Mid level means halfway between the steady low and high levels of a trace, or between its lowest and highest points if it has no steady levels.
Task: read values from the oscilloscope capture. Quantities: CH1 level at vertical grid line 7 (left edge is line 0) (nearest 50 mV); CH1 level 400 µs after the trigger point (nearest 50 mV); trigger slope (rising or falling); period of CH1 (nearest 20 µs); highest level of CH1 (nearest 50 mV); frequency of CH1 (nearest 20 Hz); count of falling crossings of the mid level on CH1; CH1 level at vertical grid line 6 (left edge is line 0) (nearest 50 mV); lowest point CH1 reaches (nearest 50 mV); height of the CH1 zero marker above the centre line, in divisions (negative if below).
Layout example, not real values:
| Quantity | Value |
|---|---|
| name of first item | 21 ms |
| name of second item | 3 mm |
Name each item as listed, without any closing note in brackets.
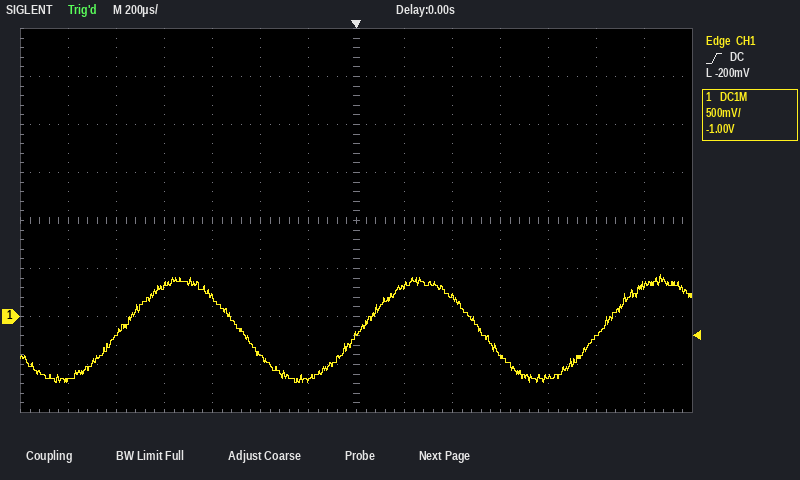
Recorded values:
| Quantity | Value |
|---|---|
| CH1 level at vertical grid line 7 (left edge is line 0) | -200 mV |
| CH1 level 400 µs after the trigger point | 200 mV |
| trigger slope | rising |
| period of CH1 | 1.00 ms |
| highest level of CH1 | 450 mV |
| frequency of CH1 | 1.00 kHz |
| count of falling crossings of the mid level on CH1 | 2 |
| CH1 level at vertical grid line 6 (left edge is line 0) | -650 mV |
| lowest point CH1 reaches | -700 mV |
| height of the CH1 zero marker above the centre line, in divisions | -2.0 div |
